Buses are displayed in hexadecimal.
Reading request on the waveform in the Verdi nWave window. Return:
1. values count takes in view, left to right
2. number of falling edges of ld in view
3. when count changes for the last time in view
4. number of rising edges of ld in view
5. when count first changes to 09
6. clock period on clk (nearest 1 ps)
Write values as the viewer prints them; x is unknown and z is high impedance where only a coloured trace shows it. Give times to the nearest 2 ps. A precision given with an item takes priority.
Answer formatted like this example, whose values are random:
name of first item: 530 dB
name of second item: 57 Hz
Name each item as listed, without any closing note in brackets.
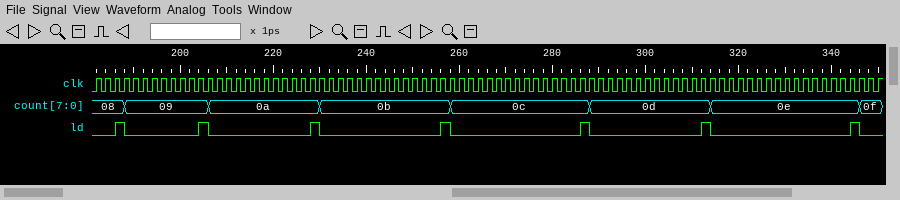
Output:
values count takes in view, left to right: 08, 09, 0a, 0b, 0c, 0d, 0e, 0f
number of falling edges of ld in view: 7
when count changes for the last time in view: 346 ps
number of rising edges of ld in view: 7
when count first changes to 09: 188 ps
clock period on clk: 2 ps
